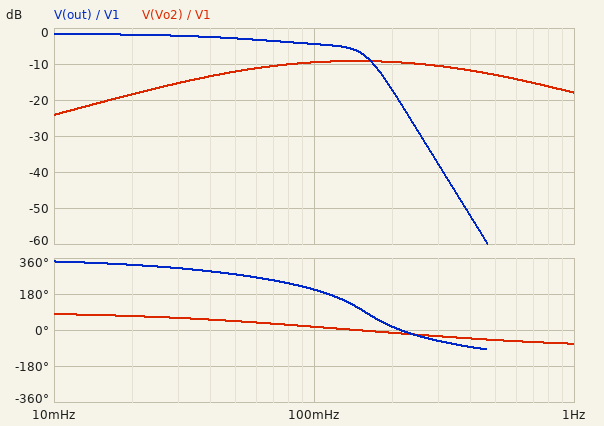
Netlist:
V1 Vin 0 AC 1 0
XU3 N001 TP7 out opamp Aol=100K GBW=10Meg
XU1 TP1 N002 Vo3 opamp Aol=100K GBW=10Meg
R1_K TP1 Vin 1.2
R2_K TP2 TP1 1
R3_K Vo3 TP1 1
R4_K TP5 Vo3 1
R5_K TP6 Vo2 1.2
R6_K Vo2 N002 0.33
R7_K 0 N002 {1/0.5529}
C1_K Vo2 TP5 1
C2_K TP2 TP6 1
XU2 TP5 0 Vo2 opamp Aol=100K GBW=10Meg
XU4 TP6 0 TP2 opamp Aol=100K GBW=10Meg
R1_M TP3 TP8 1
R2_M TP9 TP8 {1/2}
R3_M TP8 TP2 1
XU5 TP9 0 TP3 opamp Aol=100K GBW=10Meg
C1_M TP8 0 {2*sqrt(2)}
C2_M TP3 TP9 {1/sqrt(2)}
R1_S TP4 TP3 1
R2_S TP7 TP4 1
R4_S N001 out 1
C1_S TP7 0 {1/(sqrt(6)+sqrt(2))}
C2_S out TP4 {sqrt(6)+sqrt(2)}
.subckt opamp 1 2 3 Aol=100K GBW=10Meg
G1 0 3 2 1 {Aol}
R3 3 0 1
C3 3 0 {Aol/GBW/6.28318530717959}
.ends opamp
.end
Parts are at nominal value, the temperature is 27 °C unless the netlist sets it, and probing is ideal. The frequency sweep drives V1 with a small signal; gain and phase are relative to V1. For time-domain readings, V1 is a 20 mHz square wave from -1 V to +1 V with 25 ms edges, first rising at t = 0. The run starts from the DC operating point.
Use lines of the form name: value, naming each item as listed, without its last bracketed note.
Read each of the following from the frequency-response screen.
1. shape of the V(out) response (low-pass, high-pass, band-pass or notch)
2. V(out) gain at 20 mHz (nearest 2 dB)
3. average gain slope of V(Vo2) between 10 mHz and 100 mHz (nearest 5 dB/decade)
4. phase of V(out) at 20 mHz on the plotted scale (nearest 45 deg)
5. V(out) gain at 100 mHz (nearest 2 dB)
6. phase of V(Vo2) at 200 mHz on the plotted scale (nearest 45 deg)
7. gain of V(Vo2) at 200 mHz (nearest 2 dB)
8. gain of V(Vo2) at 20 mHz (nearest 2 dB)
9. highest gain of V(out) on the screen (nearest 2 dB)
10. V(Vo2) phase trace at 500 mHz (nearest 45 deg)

shape of the V(out) response: low-pass
V(out) gain at 20 mHz: -2 dB
average gain slope of V(Vo2) between 10 mHz and 100 mHz: 15 dB/decade
phase of V(out) at 20 mHz on the plotted scale: 315 deg
V(out) gain at 100 mHz: -4 dB
phase of V(Vo2) at 200 mHz on the plotted scale: 0 deg
gain of V(Vo2) at 200 mHz: -10 dB
gain of V(Vo2) at 20 mHz: -18 dB
highest gain of V(out) on the screen: -2 dB
V(Vo2) phase trace at 500 mHz: -45 deg
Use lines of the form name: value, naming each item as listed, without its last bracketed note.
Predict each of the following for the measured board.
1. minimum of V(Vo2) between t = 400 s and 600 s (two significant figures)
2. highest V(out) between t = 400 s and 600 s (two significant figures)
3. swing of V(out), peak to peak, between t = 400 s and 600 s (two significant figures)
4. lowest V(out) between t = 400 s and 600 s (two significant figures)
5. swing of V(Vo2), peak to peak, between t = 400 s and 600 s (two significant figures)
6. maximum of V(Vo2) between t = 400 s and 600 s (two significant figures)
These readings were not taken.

minimum of V(Vo2) between t = 400 s and 600 s: -560 mV
highest V(out) between t = 400 s and 600 s: 850 mV
swing of V(out), peak to peak, between t = 400 s and 600 s: 1.7 V
lowest V(out) between t = 400 s and 600 s: -850 mV
swing of V(Vo2), peak to peak, between t = 400 s and 600 s: 1.1 V
maximum of V(Vo2) between t = 400 s and 600 s: 560 mV
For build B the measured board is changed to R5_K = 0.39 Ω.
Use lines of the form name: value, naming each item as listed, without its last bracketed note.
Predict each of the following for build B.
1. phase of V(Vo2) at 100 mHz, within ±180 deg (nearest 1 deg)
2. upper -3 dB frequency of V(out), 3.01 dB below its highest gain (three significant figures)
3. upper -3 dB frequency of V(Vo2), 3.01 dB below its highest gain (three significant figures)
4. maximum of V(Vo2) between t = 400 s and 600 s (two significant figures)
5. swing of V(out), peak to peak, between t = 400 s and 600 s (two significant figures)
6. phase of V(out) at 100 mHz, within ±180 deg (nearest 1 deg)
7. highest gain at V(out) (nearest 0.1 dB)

phase of V(Vo2) at 100 mHz, within ±180 deg: 55 deg
upper -3 dB frequency of V(out), 3.01 dB below its highest gain: 169 mHz
upper -3 dB frequency of V(Vo2), 3.01 dB below its highest gain: 509 mHz
maximum of V(Vo2) between t = 400 s and 600 s: 460 mV
swing of V(out), peak to peak, between t = 400 s and 600 s: 2.7 V
phase of V(out) at 100 mHz, within ±180 deg: -119 deg
highest gain at V(out): 1.7 dB
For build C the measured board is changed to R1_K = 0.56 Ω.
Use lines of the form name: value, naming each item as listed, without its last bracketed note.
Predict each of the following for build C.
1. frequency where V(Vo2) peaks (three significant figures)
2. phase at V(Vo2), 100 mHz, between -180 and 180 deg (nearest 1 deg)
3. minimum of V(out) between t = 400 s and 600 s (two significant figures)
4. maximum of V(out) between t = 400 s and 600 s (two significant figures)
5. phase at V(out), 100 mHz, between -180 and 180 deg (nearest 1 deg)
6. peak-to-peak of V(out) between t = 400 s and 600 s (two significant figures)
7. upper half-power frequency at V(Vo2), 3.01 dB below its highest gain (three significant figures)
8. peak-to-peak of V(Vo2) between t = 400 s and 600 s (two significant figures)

frequency where V(Vo2) peaks: 145 mHz
phase at V(Vo2), 100 mHz, between -180 and 180 deg: 12 deg
minimum of V(out) between t = 400 s and 600 s: -1.8 V
maximum of V(out) between t = 400 s and 600 s: 1.8 V
phase at V(out), 100 mHz, between -180 and 180 deg: -162 deg
peak-to-peak of V(out) between t = 400 s and 600 s: 3.6 V
upper half-power frequency at V(Vo2), 3.01 dB below its highest gain: 548 mHz
peak-to-peak of V(Vo2) between t = 400 s and 600 s: 1.9 V
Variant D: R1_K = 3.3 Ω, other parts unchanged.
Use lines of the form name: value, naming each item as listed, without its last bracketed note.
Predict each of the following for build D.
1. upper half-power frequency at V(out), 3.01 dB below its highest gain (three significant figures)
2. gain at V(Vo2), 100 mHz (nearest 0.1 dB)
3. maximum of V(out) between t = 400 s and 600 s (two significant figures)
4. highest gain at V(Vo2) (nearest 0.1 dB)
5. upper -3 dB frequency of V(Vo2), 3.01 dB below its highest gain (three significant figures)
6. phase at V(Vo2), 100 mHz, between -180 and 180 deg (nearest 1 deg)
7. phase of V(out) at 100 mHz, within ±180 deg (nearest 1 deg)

upper half-power frequency at V(out), 3.01 dB below its highest gain: 147 mHz
gain at V(Vo2), 100 mHz: -16.7 dB
maximum of V(out) between t = 400 s and 600 s: 350 mV
highest gain at V(Vo2): -16.2 dB
upper -3 dB frequency of V(Vo2), 3.01 dB below its highest gain: 367 mHz
phase at V(Vo2), 100 mHz, between -180 and 180 deg: 20 deg
phase of V(out) at 100 mHz, within ±180 deg: -154 deg
